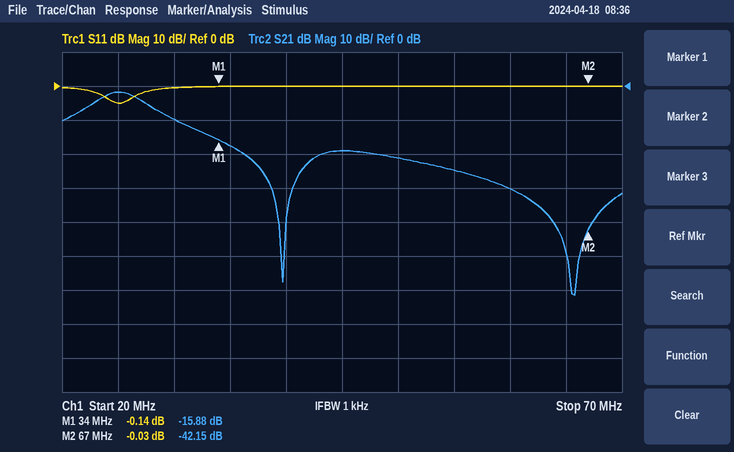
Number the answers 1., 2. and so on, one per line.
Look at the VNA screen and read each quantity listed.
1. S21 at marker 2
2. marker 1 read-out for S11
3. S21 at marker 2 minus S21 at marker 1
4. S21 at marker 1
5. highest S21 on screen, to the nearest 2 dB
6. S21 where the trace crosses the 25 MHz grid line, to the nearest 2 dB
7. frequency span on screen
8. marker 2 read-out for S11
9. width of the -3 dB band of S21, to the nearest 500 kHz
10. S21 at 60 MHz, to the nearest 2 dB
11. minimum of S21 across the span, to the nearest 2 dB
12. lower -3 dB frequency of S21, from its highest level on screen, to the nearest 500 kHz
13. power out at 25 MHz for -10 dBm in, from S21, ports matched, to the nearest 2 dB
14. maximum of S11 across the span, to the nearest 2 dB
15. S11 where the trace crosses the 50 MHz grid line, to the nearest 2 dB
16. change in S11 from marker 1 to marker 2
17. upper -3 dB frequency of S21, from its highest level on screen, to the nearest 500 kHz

1. -42.15 dB
2. -0.14 dB
3. -26.27 dB
4. -15.88 dB
5. -2 dB
6. -2 dB
7. 50 MHz
8. -0.03 dB
9. 4.5 MHz
10. -30 dB
11. -62 dB
12. 23.0 MHz
13. -12 dBm
14. 0 dB
15. 0 dB
16. 0.11 dB
17. 27.5 MHz
